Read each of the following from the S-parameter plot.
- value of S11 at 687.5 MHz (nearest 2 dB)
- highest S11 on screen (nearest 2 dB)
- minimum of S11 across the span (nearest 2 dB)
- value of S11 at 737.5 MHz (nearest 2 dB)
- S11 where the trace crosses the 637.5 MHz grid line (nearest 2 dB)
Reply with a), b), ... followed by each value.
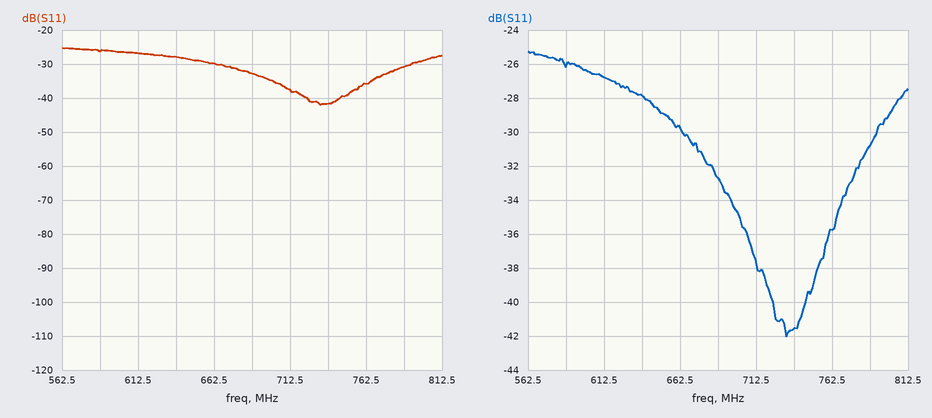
a) -32 dB
b) -26 dB
c) -42 dB
d) -42 dB
e) -28 dB
